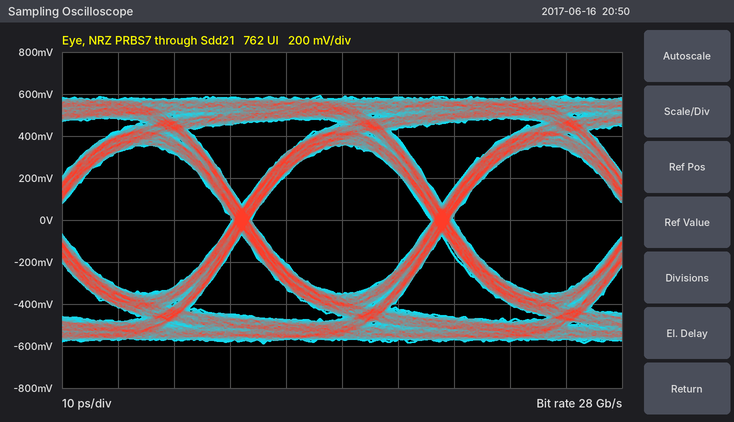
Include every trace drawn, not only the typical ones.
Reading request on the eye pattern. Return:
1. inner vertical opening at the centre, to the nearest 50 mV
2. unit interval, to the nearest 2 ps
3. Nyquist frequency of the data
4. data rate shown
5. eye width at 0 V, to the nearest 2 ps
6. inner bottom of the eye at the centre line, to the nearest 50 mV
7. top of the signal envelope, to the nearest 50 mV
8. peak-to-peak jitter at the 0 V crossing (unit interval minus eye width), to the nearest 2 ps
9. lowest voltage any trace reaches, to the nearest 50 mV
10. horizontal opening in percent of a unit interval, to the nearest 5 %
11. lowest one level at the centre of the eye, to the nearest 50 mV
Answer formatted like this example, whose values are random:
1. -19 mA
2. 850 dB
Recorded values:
1. 700 mV
2. 36 ps
3. 14 GHz
4. 28 Gb/s
5. 32 ps
6. -350 mV
7. 600 mV
8. 4 ps
9. -600 mV
10. 90 %
11. 350 mV
